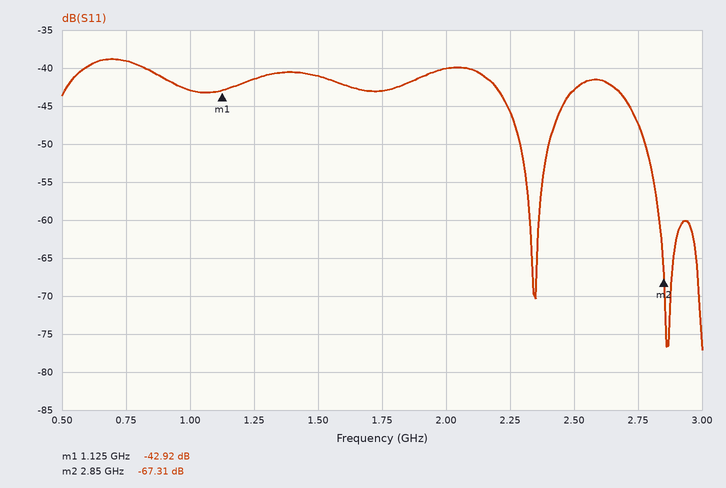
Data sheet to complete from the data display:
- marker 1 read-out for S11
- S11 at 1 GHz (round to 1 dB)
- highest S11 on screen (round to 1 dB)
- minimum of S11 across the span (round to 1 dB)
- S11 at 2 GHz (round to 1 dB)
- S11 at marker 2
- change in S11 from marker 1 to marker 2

-42.92 dB
-43 dB
-39 dB
-77 dB
-40 dB
-67.31 dB
-24.39 dB
